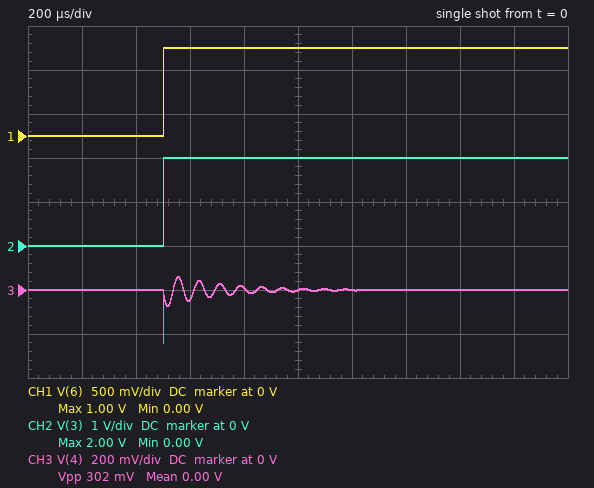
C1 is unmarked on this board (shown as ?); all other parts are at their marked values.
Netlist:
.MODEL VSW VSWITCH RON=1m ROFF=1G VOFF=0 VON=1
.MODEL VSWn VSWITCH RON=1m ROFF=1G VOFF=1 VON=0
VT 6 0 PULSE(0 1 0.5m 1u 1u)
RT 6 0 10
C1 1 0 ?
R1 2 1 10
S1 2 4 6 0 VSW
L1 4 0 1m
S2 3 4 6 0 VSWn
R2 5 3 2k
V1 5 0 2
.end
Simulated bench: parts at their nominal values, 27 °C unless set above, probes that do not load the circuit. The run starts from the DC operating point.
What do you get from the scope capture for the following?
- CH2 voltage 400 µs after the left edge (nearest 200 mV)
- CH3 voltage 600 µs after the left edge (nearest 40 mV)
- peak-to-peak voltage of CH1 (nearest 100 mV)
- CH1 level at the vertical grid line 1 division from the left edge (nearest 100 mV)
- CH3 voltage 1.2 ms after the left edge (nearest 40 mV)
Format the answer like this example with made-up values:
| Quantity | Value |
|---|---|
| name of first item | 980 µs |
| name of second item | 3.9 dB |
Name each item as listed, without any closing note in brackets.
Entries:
| Quantity | Value |
|---|---|
| CH2 voltage 400 µs after the left edge | 0 V |
| CH3 voltage 600 µs after the left edge | -40 mV |
| peak-to-peak voltage of CH1 | 1.0 V |
| CH1 level at the vertical grid line 1 division from the left edge | 0 V |
| CH3 voltage 1.2 ms after the left edge | 0 V |
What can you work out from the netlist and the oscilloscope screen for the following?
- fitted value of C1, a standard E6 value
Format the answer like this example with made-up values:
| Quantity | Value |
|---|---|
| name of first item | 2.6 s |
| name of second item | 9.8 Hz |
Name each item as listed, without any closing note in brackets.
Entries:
| Quantity | Value |
|---|---|
| fitted value of C1, a standard E6 value | 150 nF |
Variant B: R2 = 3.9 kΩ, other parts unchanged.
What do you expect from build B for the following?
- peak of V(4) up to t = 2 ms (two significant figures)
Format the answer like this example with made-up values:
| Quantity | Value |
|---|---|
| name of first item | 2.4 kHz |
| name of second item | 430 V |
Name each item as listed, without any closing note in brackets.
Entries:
| Quantity | Value |
|---|---|
| peak of V(4) up to t = 2 ms | 31 mV |
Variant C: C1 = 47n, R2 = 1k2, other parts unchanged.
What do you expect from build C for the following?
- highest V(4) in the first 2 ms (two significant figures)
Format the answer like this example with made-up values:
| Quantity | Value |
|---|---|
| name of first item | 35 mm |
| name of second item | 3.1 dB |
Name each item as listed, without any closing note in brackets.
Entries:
| Quantity | Value |
|---|---|
| highest V(4) in the first 2 ms | 200 mV |
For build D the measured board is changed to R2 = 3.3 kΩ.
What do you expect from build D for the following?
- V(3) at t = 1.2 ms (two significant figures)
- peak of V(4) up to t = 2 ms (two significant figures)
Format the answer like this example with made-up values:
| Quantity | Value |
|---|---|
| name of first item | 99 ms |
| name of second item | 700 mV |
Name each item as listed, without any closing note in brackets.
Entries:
| Quantity | Value |
|---|---|
| V(3) at t = 1.2 ms | 2.0 V |
| peak of V(4) up to t = 2 ms | 37 mV |
